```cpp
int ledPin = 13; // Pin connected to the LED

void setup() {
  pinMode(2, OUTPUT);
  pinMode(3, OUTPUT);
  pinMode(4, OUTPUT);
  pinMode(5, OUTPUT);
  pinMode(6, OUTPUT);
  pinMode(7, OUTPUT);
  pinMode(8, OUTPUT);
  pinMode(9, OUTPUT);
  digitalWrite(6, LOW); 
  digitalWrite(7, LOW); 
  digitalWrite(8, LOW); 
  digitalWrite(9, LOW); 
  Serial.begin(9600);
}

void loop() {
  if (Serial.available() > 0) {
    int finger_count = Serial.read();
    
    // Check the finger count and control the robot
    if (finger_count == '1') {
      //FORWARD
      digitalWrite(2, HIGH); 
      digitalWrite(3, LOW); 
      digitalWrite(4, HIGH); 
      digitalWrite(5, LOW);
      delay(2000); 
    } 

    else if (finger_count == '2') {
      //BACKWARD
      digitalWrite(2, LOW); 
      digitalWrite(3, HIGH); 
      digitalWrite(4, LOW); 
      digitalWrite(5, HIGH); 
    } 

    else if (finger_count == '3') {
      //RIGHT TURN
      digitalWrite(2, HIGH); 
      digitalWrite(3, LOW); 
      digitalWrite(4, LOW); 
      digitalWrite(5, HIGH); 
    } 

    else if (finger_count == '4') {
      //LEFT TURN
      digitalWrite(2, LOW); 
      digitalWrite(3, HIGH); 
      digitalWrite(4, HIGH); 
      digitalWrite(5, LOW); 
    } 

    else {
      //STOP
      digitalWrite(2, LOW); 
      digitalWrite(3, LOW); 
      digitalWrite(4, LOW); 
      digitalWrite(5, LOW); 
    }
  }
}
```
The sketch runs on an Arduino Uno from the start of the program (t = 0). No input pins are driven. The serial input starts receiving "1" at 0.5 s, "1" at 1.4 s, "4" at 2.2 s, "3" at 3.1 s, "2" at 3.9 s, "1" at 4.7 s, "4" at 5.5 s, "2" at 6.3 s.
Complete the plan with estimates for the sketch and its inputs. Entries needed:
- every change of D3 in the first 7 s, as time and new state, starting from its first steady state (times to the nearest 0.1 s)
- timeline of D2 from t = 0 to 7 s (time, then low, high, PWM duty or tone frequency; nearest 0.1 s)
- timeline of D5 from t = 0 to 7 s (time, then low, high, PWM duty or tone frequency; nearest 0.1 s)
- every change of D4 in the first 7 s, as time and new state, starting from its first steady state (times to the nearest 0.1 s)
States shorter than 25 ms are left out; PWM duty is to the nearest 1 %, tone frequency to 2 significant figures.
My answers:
0 s low; 4.5 s high; 4.7 s low; 6.7 s high
0 s low; 0.5 s high; 4.5 s low; 4.7 s high; 6.7 s low
0 s low; 4.5 s high; 4.7 s low; 6.7 s high
0 s low; 0.5 s high; 4.5 s low; 4.7 s high; 6.7 s low
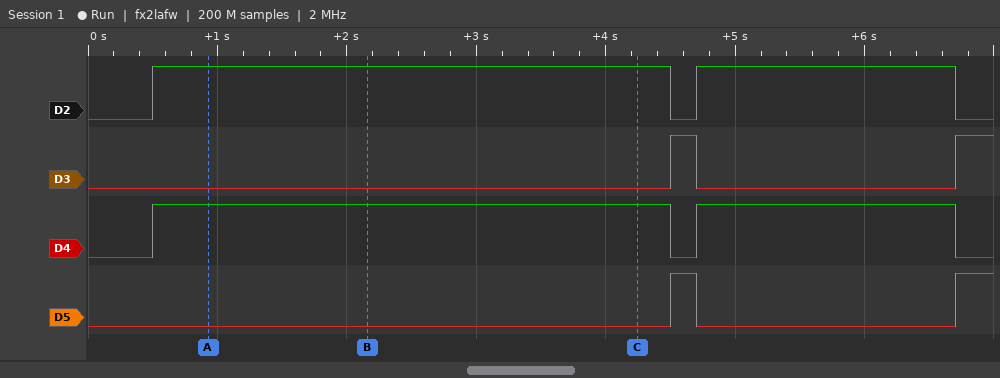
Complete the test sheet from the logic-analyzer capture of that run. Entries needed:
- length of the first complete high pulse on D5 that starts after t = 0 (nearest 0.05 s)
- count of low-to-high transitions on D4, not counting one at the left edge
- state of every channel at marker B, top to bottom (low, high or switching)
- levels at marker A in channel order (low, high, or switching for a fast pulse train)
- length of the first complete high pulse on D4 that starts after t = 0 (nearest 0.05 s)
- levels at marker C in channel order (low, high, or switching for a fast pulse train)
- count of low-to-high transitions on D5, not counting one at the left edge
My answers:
0.20 s
2
D2 high, D3 low, D4 high, D5 low
D2 high, D3 low, D4 high, D5 low
4.00 s
D2 high, D3 low, D4 high, D5 low
2
